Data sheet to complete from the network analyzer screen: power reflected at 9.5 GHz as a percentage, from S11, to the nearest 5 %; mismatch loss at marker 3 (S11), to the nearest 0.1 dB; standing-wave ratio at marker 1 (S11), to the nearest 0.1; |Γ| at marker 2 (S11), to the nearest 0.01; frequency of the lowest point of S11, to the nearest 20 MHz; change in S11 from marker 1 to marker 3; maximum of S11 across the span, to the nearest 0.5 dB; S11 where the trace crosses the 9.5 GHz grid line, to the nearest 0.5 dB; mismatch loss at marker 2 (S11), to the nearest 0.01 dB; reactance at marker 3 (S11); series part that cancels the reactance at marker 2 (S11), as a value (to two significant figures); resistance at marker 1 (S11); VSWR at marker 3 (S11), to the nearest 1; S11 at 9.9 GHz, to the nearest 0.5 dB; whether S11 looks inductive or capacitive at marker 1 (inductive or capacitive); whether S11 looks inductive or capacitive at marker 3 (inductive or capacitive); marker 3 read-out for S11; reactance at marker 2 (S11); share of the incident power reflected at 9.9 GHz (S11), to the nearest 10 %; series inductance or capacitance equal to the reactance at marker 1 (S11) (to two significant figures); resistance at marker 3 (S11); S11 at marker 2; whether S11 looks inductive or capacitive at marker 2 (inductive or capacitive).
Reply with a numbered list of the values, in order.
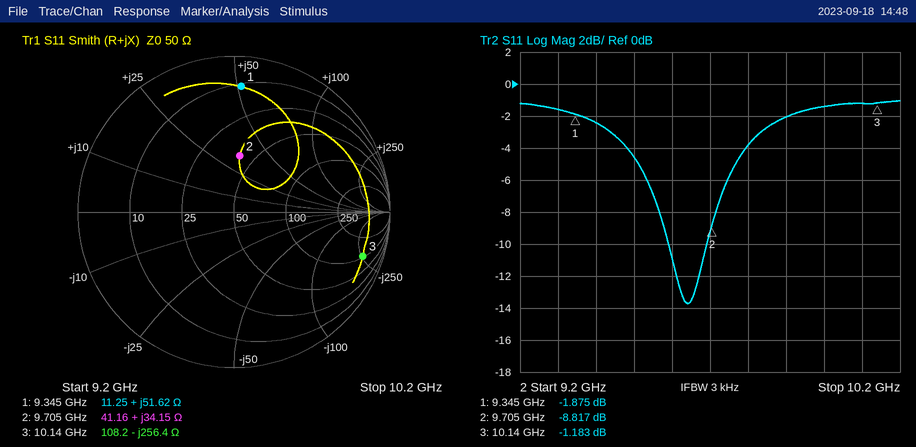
1. 35 %
2. 6.2 dB
3. 9.3
4. 0.36
5. 9.64 GHz
6. 0.692 dB
7. -1.0 dB
8. -4.5 dB
9. 0.61 dB
10. -256.4 Ω
11. 480 fF
12. 11.25 Ω
13. 15
14. -2.0 dB
15. inductive
16. capacitive
17. -1.183 dB
18. +34.15 Ω
19. 60 %
20. 880 pH
21. 108.2 Ω
22. -8.817 dB
23. inductive
